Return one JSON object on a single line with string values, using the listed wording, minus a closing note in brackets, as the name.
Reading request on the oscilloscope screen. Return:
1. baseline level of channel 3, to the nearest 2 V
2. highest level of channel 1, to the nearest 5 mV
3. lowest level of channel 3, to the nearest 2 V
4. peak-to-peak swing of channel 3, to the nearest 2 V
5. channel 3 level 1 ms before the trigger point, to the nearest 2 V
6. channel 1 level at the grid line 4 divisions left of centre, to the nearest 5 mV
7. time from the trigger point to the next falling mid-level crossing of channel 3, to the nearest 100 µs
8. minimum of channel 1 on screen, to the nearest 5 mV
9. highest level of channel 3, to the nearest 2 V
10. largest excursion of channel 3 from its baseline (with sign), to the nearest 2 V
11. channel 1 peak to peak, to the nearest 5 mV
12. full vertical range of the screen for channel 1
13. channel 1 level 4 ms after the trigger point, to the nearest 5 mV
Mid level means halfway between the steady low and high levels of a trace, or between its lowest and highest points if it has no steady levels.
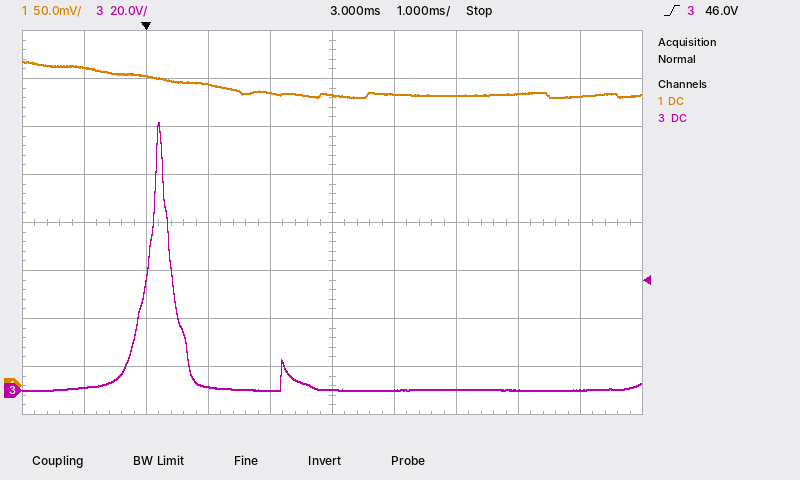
{"baseline level of channel 3, to the nearest 2 V": "0 V", "highest level of channel 1, to the nearest 5 mV": "340 mV", "lowest level of channel 3, to the nearest 2 V": "0 V", "peak-to-peak swing of channel 3, to the nearest 2 V": "112 V", "channel 3 level 1 ms before the trigger point, to the nearest 2 V": "2 V", "channel 1 level at the grid line 4 divisions left of centre, to the nearest 5 mV": "330 mV", "time from the trigger point to the next falling mid-level crossing of channel 3, to the nearest 100 µs": "400 µs", "minimum of channel 1 on screen, to the nearest 5 mV": "300 mV", "highest level of channel 3, to the nearest 2 V": "112 V", "largest excursion of channel 3 from its baseline (with sign), to the nearest 2 V": "+112 V", "channel 1 peak to peak, to the nearest 5 mV": "40 mV", "full vertical range of the screen for channel 1": "400 mV", "channel 1 level 4 ms after the trigger point, to the nearest 5 mV": "305 mV"}
